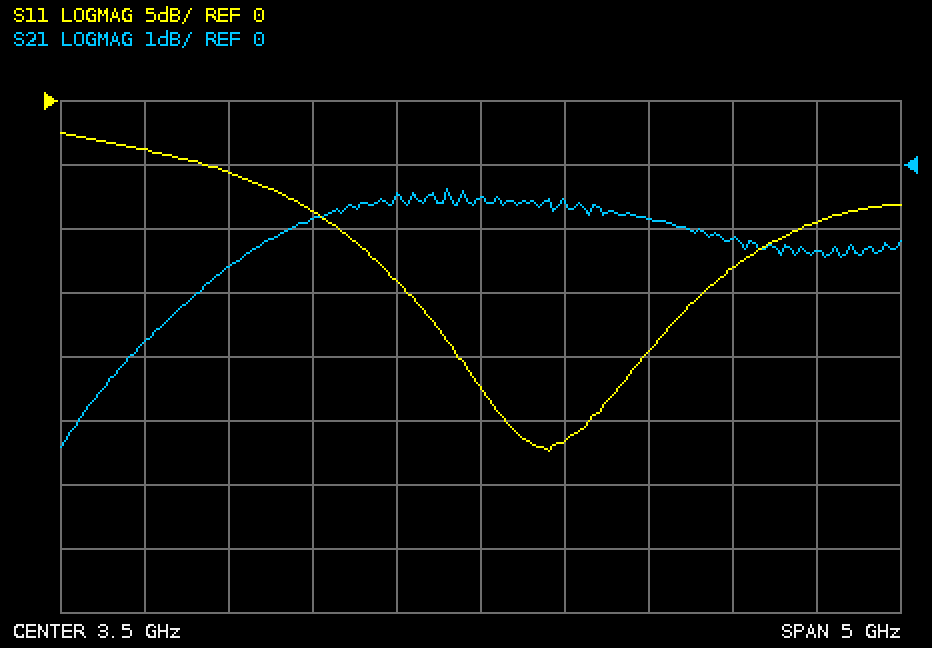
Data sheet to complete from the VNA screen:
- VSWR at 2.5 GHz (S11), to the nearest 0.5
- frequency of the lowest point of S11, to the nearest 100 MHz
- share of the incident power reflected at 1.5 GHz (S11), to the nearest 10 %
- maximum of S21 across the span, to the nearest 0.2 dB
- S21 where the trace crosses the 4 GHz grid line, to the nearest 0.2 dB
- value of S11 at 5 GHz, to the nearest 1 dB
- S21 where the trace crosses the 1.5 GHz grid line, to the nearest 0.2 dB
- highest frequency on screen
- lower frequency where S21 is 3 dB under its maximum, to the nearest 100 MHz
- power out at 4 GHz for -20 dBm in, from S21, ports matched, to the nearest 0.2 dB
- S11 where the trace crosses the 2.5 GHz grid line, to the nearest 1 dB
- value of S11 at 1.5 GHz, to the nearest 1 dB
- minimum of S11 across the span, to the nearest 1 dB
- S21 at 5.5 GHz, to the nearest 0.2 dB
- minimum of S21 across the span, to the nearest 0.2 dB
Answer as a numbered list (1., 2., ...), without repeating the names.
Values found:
1. 2.0
2. 3.9 GHz
3. 40 %
4. -0.4 dB
5. -0.6 dB
6. -13 dB
7. -2.8 dB
8. 6 GHz
9. 1.3 GHz
10. -20.6 dBm
11. -9 dB
12. -4 dB
13. -27 dB
14. -1.4 dB
15. -4.4 dB
